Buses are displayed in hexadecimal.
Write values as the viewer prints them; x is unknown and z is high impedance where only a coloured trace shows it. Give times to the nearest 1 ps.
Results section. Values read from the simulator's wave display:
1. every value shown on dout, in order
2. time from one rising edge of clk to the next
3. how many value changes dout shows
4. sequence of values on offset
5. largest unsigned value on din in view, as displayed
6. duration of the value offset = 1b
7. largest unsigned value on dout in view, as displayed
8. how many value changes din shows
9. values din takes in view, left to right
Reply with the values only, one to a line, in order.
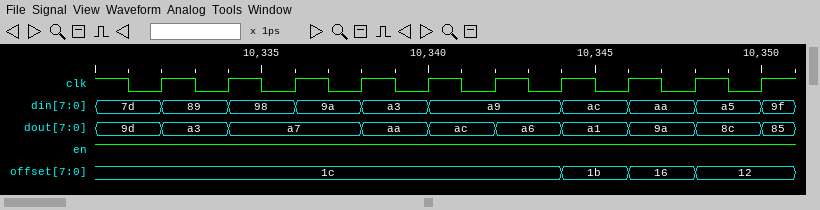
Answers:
9d, a3, a7, aa, ac, a6, a1, 9a, 8c, 85
2 ps
9
1c, 1b, 16, 12
ac
2 ps
ac
9
7d, 89, 98, 9a, a3, a9, ac, aa, a5, 9f
